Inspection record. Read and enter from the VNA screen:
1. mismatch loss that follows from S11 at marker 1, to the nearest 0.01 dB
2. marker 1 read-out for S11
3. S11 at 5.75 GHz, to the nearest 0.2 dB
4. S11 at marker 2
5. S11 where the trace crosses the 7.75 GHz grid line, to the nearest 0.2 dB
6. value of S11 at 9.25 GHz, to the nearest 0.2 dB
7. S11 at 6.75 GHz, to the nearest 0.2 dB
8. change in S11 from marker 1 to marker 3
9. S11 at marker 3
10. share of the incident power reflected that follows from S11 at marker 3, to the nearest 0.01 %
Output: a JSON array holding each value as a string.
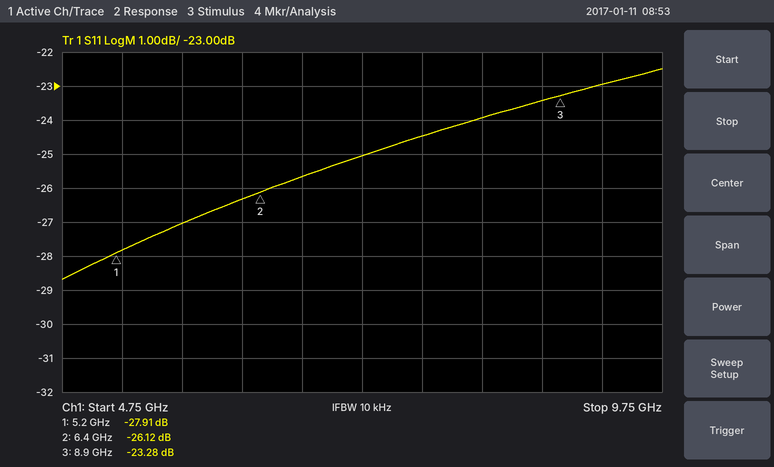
["0.01 dB", "-27.91 dB", "-27.0 dB", "-26.12 dB", "-24.4 dB", "-23.0 dB", "-25.6 dB", "4.63 dB", "-23.28 dB", "0.47 %"]
